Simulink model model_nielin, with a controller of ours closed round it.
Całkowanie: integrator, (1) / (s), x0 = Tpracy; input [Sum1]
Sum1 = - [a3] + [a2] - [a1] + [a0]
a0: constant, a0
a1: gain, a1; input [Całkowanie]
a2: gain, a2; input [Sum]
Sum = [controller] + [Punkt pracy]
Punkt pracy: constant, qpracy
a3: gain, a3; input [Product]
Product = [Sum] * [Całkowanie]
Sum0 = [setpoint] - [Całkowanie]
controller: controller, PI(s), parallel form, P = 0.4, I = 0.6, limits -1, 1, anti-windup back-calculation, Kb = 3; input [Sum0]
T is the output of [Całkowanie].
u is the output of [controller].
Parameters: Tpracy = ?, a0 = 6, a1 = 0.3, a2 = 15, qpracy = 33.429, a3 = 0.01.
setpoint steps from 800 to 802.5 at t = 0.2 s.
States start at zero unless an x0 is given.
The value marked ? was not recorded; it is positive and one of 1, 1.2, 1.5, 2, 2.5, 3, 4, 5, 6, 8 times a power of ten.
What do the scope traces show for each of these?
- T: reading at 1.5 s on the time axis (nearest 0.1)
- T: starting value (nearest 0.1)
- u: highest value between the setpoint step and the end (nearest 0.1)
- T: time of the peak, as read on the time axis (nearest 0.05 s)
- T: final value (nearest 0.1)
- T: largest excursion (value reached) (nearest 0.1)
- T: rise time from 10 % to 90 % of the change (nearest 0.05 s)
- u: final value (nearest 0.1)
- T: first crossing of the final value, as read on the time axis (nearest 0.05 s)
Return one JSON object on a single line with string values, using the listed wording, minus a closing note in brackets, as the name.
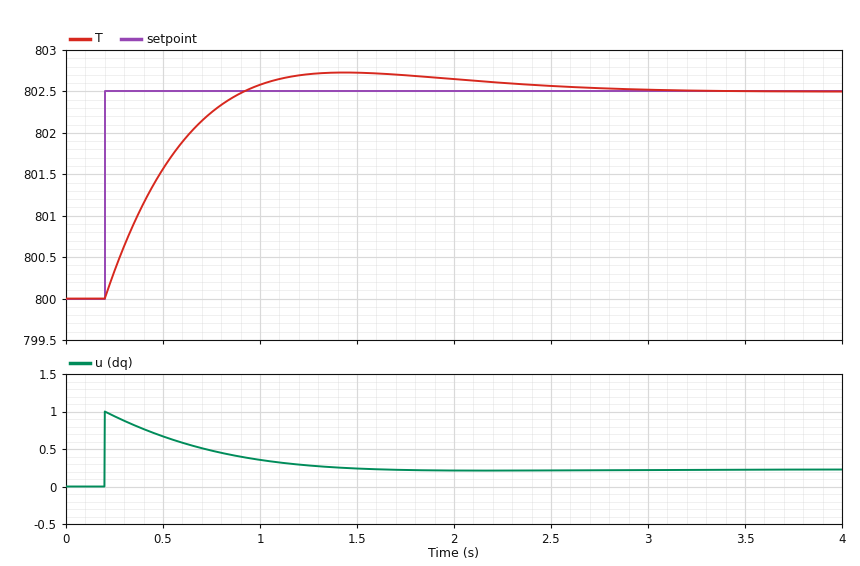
{"T: reading at 1.5 s on the time axis": "802.7", "T: starting value": "800.0", "u: highest value between the setpoint step and the end": "1.0", "T: time of the peak, as read on the time axis": "1.45 s", "T: final value": "802.5", "T: largest excursion (value reached)": "802.7", "T: rise time from 10 % to 90 % of the change": "0.50 s", "u: final value": "0.2", "T: first crossing of the final value, as read on the time axis": "0.90 s"}
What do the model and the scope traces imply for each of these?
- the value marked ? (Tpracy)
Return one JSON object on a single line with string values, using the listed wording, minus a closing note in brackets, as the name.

{"the value marked ?": "800"}
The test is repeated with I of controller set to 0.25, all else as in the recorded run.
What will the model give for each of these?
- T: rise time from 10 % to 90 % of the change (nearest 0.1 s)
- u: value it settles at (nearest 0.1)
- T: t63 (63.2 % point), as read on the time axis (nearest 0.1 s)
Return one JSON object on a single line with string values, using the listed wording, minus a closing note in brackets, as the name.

{"T: rise time from 10 % to 90 % of the change": "0.8 s", "u: value it settles at": "0.2", "T: t63 (63.2 % point), as read on the time axis": "0.6 s"}
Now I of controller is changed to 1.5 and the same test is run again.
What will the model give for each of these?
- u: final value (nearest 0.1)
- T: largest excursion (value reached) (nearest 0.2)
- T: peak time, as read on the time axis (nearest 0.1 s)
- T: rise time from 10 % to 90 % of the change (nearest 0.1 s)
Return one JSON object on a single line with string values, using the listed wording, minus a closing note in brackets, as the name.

{"u: final value": "0.2", "T: largest excursion (value reached)": "803.0", "T: peak time, as read on the time axis": "1.0 s", "T: rise time from 10 % to 90 % of the change": "0.3 s"}
